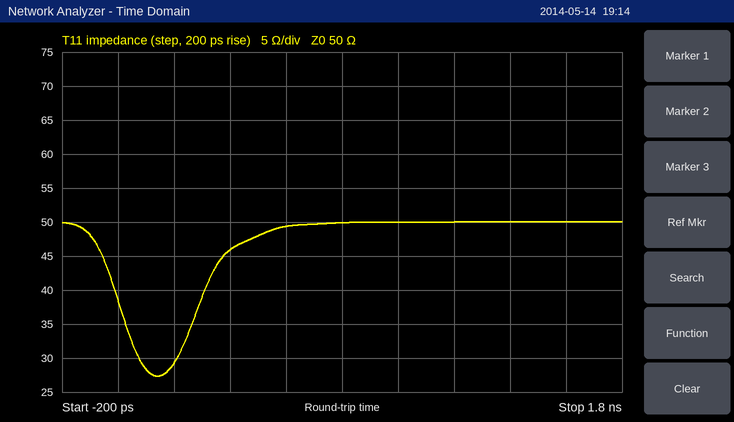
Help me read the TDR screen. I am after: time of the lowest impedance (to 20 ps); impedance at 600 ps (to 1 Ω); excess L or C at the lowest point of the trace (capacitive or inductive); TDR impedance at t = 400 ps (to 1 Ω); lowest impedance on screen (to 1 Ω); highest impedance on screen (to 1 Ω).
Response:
140 ps
49 Ω
capacitive
46 Ω
27 Ω
50 Ω
